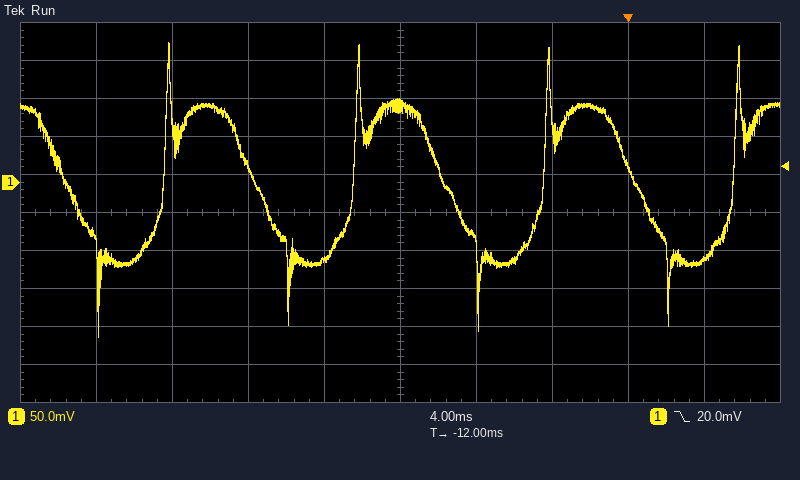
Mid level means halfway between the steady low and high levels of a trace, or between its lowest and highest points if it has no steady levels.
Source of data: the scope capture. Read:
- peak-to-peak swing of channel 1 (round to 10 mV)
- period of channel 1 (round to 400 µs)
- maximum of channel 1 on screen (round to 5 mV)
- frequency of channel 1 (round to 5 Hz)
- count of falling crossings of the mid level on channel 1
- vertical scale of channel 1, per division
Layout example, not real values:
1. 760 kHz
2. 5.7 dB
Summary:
1. 390 mV
2. 10.0 ms
3. 185 mV
4. 100 Hz
5. 4
6. 50 mV
